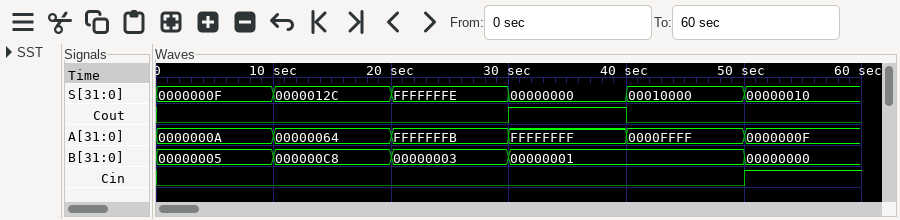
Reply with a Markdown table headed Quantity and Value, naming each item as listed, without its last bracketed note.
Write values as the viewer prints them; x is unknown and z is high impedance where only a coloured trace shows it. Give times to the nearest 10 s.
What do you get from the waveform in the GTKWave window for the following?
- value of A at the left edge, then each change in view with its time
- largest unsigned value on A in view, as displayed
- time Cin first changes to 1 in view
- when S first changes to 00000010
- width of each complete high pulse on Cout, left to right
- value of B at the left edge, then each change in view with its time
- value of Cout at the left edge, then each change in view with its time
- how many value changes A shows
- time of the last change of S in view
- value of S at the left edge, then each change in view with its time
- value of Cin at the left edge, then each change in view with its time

| Quantity | Value |
|---|---|
| value of A at the left edge, then each change in view with its time | 0000000A, 00000064 at 10 s, FFFFFFFB at 20 s, FFFFFFFF at 30 s, 0000FFFF at 40 s, 0000000F at 50 s |
| largest unsigned value on A in view, as displayed | FFFFFFFF |
| time Cin first changes to 1 in view | 50 s |
| when S first changes to 00000010 | 50 s |
| width of each complete high pulse on Cout, left to right | 10 s |
| value of B at the left edge, then each change in view with its time | 00000005, 000000C8 at 10 s, 00000003 at 20 s, 00000001 at 30 s, 00000000 at 50 s |
| value of Cout at the left edge, then each change in view with its time | 0, 1 at 30 s, 0 at 40 s |
| how many value changes A shows | 5 |
| time of the last change of S in view | 50 s |
| value of S at the left edge, then each change in view with its time | 0000000F, 0000012C at 10 s, FFFFFFFE at 20 s, 00000000 at 30 s, 00010000 at 40 s, 00000010 at 50 s |
| value of Cin at the left edge, then each change in view with its time | 0, 1 at 50 s |
